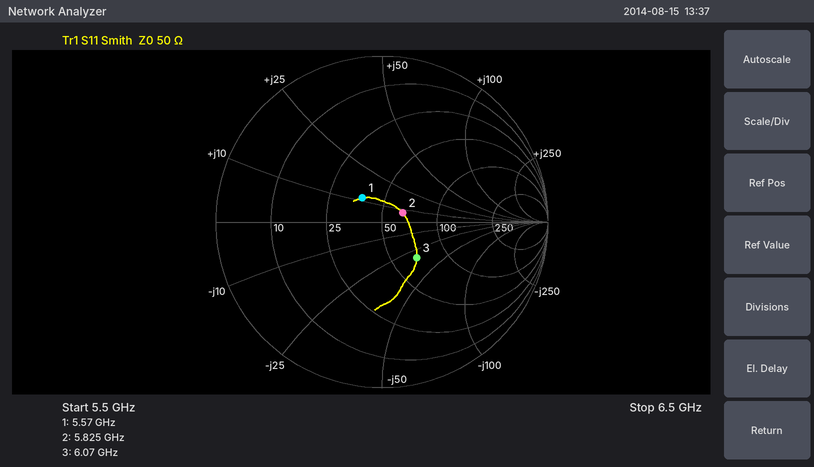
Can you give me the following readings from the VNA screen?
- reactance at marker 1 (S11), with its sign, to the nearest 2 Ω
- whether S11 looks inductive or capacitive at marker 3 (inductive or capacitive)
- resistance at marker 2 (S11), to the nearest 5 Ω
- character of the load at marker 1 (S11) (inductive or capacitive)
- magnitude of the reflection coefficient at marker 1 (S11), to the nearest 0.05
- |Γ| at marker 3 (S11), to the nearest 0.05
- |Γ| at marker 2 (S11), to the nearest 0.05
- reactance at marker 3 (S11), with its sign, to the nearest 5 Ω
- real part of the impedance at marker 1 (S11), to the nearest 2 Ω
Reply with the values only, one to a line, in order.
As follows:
+12 Ω
capacitive
65 Ω
inductive
0.20
0.30
0.15
-30 Ω
38 Ω
